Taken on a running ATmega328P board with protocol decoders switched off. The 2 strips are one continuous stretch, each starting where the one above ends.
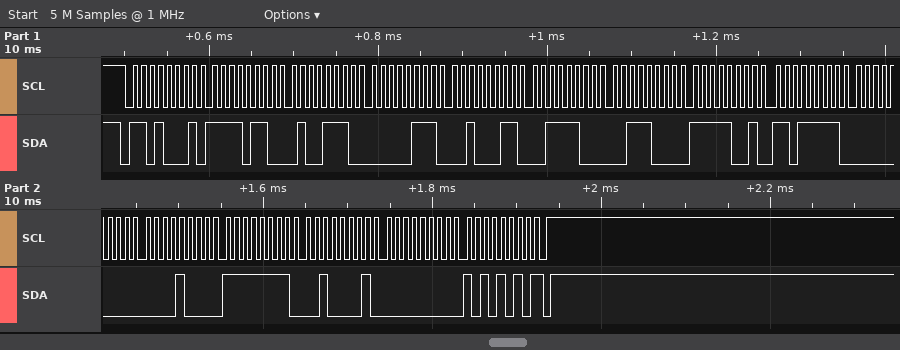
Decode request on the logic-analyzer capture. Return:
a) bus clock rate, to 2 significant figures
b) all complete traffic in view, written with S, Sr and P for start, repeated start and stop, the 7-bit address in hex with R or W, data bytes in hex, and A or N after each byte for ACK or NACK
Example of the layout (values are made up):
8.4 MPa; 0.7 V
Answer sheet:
100 kHz; S 68R A F6 A 4E A 07 A 23 A 3C A 38 A F9 A DF A 00 A 08 A FF A 21 A 00 A AA N P
